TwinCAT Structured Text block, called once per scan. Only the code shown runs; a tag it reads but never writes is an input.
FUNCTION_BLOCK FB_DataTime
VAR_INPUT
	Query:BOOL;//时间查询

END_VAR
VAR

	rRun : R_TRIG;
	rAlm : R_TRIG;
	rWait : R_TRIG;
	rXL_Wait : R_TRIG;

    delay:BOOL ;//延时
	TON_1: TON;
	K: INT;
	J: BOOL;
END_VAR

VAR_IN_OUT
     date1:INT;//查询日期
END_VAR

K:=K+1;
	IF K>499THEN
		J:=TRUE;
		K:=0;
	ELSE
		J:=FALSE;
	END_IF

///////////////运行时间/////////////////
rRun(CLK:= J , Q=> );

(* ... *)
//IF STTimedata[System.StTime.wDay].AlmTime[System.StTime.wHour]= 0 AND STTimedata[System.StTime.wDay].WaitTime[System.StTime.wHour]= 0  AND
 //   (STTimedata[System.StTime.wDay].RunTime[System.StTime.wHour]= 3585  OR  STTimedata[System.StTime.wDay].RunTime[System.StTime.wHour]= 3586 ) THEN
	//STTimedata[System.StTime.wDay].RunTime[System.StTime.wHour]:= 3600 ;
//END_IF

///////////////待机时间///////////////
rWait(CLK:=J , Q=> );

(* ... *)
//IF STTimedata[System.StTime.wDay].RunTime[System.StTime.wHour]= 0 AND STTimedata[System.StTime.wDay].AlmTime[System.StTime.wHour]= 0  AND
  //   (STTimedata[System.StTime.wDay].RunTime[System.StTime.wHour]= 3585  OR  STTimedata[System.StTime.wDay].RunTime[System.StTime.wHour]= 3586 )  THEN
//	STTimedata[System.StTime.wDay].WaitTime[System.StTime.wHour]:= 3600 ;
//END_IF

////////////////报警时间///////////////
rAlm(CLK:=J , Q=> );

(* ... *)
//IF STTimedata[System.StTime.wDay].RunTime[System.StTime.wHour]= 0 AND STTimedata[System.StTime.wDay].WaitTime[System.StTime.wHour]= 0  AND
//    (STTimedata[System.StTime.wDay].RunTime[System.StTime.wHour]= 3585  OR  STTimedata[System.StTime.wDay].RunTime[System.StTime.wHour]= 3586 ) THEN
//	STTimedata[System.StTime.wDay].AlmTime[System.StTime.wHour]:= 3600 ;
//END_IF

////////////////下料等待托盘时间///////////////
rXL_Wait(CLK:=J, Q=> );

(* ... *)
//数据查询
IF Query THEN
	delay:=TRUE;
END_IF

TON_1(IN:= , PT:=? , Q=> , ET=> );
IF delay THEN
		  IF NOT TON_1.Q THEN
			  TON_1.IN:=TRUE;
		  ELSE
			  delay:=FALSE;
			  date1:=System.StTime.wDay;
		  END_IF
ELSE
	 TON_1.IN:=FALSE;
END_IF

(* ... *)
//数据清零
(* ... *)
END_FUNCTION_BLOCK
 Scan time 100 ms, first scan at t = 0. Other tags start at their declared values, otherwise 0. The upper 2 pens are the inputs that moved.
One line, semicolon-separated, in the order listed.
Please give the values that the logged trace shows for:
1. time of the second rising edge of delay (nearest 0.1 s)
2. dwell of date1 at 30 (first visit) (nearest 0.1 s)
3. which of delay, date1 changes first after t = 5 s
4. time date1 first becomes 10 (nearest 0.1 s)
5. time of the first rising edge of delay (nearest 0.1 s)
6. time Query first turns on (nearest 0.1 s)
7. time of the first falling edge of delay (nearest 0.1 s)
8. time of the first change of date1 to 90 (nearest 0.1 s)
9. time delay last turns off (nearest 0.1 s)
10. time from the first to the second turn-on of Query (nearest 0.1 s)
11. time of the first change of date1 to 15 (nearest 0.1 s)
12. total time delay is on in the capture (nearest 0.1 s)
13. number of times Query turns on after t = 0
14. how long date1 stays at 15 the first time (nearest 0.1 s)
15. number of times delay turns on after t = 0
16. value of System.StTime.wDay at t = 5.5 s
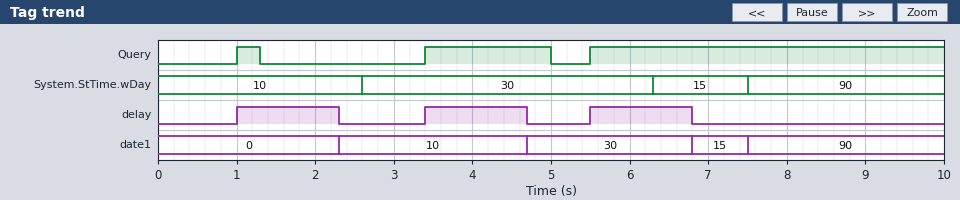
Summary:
3.4 s; 2.1 s; delay; 2.3 s; 1.0 s; 1.0 s; 2.3 s; 7.5 s; 6.8 s; 2.4 s; 6.8 s; 3.9 s; 3; 0.7 s; 3; 30
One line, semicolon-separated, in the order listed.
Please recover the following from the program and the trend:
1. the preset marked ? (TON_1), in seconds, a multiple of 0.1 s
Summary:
1.2 s
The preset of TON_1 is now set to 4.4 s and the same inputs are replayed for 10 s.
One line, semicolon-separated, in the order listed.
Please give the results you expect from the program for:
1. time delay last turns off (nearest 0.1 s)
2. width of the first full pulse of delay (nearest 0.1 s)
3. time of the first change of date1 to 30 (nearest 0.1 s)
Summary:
5.5 s; 4.5 s; 5.5 s
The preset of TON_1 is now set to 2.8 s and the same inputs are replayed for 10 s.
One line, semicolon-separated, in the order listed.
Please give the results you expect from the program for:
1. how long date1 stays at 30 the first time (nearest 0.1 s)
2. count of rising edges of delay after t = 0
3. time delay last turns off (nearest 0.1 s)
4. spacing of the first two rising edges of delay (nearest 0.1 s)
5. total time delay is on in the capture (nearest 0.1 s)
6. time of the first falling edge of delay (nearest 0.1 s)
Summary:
4.5 s; 2; 8.4 s; 4.5 s; 5.8 s; 3.9 s
